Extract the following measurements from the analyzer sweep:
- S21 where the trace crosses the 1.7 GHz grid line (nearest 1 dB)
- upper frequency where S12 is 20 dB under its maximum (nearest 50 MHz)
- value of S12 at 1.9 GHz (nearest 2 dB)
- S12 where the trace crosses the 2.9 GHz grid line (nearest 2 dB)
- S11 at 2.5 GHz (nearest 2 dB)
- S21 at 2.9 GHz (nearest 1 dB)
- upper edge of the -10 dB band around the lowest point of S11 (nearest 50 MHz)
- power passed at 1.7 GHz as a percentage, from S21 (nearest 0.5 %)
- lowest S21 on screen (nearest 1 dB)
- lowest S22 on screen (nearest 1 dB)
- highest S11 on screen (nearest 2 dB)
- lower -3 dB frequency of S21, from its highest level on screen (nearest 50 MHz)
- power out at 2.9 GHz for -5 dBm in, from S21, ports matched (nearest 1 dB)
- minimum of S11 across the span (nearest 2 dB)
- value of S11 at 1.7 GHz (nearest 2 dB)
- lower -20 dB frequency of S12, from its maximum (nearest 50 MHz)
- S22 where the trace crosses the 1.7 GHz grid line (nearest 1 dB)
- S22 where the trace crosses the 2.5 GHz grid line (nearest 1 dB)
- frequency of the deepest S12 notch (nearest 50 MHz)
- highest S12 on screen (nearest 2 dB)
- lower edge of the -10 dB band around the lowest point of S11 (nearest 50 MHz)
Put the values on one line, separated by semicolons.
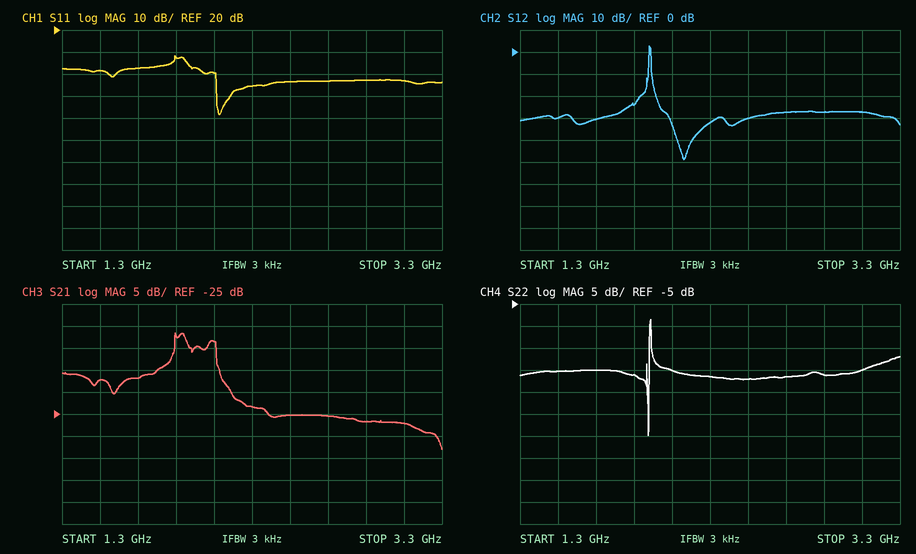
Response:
-17 dB; 2.00 GHz; -24 dB; -28 dB; -4 dB; -27 dB; 2.20 GHz; 2.0 %; -33 dB; -35 dB; 8 dB; 1.90 GHz; -32 dBm; -18 dB; 2 dB; 1.95 GHz; -20 dB; -22 dB; 2.15 GHz; 2 dB; 2.10 GHz
